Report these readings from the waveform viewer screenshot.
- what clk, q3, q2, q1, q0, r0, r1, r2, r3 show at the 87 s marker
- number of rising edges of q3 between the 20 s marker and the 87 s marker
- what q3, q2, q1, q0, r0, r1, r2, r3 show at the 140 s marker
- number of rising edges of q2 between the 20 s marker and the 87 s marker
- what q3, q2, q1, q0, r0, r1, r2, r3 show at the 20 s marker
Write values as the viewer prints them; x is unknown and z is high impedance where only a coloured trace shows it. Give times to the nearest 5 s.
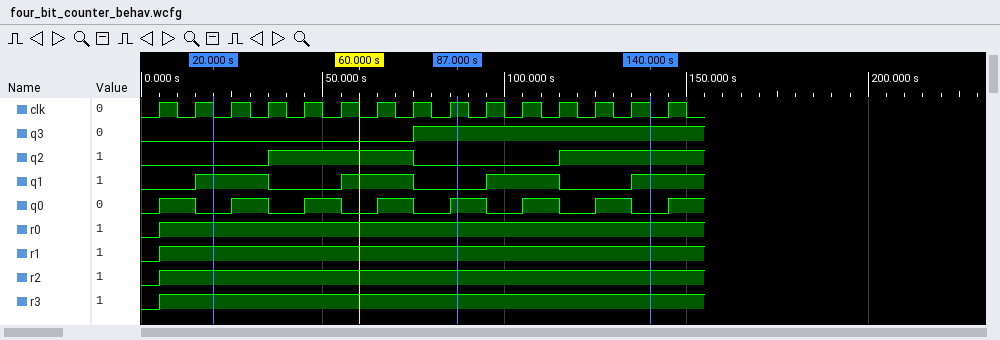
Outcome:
clk=1, q3=1, q2=0, q1=0, q0=1, r0=1, r1=1, r2=1, r3=1
1
q3=1, q2=1, q1=1, q0=0, r0=1, r1=1, r2=1, r3=1
1
q3=0, q2=0, q1=1, q0=0, r0=1, r1=1, r2=1, r3=1
